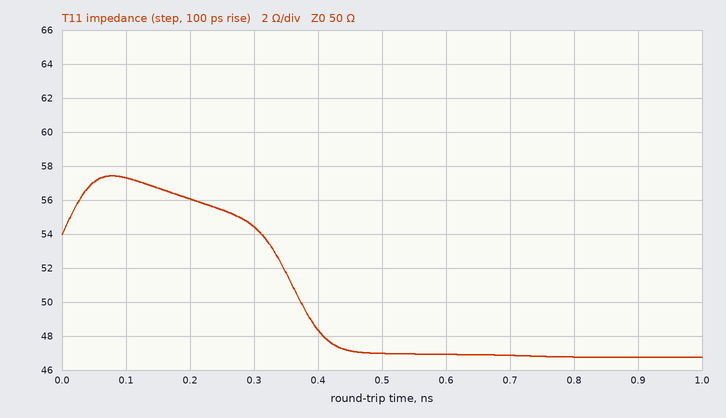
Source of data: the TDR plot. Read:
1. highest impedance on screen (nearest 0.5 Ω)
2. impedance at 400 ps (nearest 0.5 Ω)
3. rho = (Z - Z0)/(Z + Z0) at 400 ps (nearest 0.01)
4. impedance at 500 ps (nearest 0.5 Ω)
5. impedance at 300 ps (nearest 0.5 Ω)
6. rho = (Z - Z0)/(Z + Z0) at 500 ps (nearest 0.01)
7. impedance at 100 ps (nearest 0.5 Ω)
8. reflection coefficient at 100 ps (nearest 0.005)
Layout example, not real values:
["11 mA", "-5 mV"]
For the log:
["57.5 Ω", "48.5 Ω", "-0.02", "47.0 Ω", "54.5 Ω", "-0.03", "57.5 Ω", "+0.070"]
